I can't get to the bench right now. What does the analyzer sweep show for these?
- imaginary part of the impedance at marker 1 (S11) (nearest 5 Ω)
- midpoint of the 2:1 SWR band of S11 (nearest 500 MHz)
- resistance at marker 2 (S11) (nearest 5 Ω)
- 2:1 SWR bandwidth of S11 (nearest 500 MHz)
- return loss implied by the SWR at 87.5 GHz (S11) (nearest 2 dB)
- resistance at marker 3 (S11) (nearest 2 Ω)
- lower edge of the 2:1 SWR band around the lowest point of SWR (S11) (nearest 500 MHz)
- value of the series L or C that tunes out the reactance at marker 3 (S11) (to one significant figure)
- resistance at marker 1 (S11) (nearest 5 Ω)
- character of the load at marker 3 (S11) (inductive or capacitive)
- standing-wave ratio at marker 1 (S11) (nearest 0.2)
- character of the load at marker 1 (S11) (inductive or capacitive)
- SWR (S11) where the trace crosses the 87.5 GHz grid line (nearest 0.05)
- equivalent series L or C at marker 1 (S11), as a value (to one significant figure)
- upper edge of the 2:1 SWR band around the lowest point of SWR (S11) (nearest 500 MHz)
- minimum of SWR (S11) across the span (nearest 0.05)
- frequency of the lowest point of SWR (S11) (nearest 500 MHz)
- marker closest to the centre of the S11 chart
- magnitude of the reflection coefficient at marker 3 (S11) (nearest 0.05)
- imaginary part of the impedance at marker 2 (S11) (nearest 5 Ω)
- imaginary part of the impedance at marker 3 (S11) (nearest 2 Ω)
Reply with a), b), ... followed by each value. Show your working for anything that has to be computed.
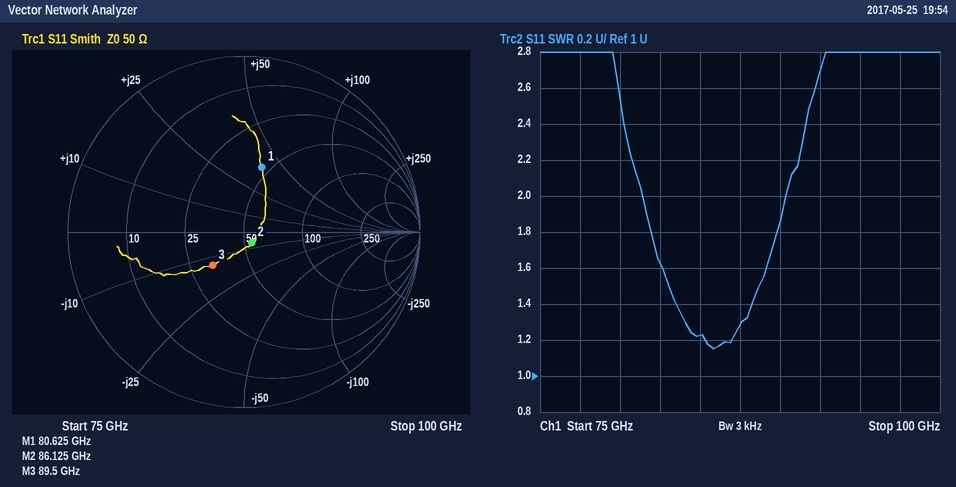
a) +40 Ω
b) 86.0 GHz
c) 55 Ω
d) 90.5 GHz − 81.5 GHz = 9.0 GHz
e) −20 log10((1.3 − 1)/(1.3 + 1)) ≈ 18 dB
f) 32 Ω
g) 81.5 GHz
h) L = 14 Ω/(2π × 89.5 GHz) ≈ 24.9 pH, so 20 pH to one significant figure
i) 45 Ω
j) capacitive
k) 2.2
l) inductive
m) 1.30
n) L = 40 Ω/(2π × 80.625 GHz) ≈ 79.0 pH, so 80 pH to one significant figure
o) 90.5 GHz
p) 1.15
q) 86.0 GHz
r) marker 2
s) 0.25
t) -5 Ω
u) -14 Ω
